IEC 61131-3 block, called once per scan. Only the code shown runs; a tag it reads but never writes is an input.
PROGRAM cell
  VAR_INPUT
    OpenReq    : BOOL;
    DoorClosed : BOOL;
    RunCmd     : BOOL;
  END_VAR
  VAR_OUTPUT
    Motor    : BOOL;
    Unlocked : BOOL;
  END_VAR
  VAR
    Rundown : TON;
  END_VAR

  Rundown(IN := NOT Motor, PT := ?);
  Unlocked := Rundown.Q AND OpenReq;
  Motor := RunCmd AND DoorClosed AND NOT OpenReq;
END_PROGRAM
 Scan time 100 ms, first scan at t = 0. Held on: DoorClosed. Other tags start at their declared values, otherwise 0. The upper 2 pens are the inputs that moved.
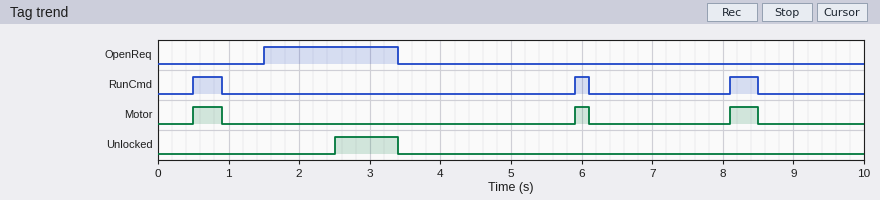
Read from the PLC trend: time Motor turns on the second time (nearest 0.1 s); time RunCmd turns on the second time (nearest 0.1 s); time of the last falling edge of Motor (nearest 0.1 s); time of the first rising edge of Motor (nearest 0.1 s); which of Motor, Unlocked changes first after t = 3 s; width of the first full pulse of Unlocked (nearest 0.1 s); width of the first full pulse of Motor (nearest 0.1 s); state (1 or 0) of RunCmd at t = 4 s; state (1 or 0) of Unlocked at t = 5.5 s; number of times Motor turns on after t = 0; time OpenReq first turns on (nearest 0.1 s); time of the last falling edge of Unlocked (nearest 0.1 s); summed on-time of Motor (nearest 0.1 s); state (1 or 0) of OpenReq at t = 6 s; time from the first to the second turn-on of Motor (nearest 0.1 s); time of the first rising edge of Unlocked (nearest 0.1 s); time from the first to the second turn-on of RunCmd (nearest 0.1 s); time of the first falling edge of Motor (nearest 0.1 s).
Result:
5.9 s
5.9 s
8.5 s
0.5 s
Unlocked
0.9 s
0.4 s
0
0
3
1.5 s
3.4 s
1.0 s
0
5.4 s
2.5 s
5.4 s
0.9 s
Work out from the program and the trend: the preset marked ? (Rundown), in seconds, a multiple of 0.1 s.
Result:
1.5 s
